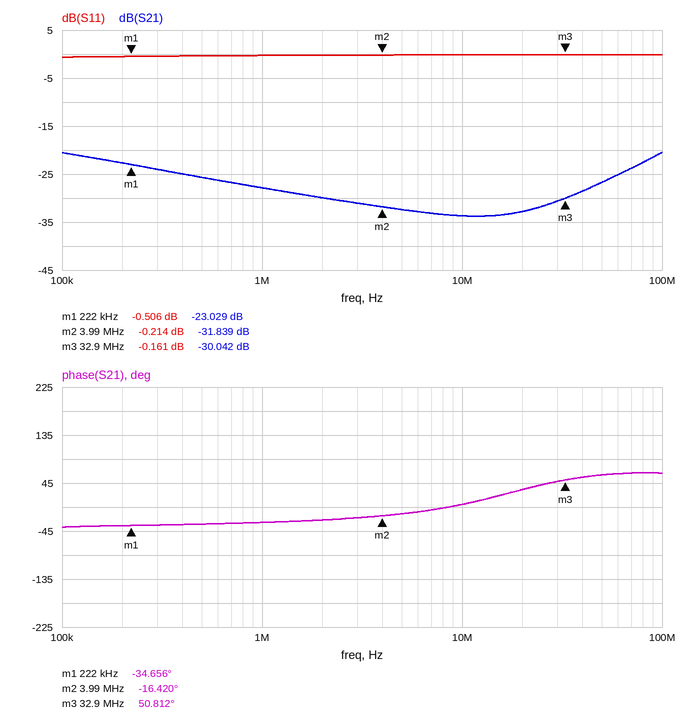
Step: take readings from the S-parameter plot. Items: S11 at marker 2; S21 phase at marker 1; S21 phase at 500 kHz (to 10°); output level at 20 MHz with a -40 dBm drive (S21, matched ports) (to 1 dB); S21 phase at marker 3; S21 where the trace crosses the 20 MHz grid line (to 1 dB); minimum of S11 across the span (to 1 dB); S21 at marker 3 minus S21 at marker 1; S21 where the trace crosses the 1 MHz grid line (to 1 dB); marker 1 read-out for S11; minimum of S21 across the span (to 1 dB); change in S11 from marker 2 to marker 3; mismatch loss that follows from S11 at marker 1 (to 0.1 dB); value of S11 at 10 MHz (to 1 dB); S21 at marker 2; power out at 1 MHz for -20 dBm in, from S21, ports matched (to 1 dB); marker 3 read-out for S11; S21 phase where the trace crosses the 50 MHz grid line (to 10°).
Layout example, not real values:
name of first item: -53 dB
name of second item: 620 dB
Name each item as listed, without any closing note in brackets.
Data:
S11 at marker 2: -0.214 dB
S21 phase at marker 1: -34.656°
S21 phase at 500 kHz: -30°
output level at 20 MHz with a -40 dBm drive (S21, matched ports): -73 dBm
S21 phase at marker 3: 50.812°
S21 where the trace crosses the 20 MHz grid line: -33 dB
minimum of S11 across the span: -1 dB
S21 at marker 3 minus S21 at marker 1: -7.013 dB
S21 where the trace crosses the 1 MHz grid line: -28 dB
marker 1 read-out for S11: -0.506 dB
minimum of S21 across the span: -34 dB
change in S11 from marker 2 to marker 3: 0.053 dB
mismatch loss that follows from S11 at marker 1: 9.6 dB
value of S11 at 10 MHz: 0 dB
S21 at marker 2: -31.839 dB
power out at 1 MHz for -20 dBm in, from S21, ports matched: -48 dBm
marker 3 read-out for S11: -0.161 dB
S21 phase where the trace crosses the 50 MHz grid line: 60°
